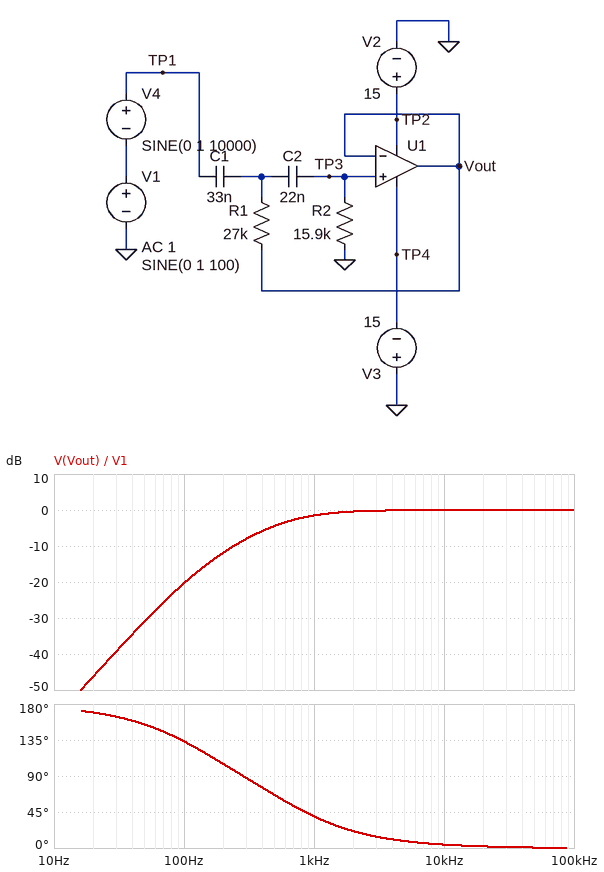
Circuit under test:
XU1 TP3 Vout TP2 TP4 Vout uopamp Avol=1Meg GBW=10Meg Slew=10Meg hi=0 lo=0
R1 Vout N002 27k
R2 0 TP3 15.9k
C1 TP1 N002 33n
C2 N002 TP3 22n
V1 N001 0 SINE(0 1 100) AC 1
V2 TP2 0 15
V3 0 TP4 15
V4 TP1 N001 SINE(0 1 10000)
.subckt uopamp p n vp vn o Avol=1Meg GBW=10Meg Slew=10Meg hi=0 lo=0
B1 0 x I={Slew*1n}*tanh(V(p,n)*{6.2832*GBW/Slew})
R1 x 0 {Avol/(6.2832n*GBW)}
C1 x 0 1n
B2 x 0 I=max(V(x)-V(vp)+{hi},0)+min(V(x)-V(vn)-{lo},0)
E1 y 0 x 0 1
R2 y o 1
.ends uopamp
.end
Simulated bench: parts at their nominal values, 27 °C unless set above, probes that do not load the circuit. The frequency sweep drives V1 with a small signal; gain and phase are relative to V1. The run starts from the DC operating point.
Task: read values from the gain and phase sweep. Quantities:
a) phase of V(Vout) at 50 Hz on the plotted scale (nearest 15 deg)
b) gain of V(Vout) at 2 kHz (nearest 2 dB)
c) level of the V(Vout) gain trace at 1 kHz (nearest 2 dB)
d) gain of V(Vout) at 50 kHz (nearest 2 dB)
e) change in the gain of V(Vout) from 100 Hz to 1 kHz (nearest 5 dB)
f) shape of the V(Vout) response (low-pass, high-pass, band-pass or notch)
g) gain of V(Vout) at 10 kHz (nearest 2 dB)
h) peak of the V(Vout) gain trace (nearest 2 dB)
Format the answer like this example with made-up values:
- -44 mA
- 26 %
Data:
- 150 deg
- 0 dB
- -2 dB
- 0 dB
- 20 dB
- high-pass
- 0 dB
- 0 dB
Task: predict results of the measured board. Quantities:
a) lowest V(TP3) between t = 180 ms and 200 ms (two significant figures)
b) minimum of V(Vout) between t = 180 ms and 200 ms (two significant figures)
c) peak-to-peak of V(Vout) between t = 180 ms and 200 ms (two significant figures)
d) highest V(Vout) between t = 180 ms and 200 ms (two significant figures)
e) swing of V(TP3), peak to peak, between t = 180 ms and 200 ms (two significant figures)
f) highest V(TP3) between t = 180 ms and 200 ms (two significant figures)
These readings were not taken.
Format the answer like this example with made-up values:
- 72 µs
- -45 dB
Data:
- -1.1 V
- -1.1 V
- 2.2 V
- 1.1 V
- 2.2 V
- 1.1 V
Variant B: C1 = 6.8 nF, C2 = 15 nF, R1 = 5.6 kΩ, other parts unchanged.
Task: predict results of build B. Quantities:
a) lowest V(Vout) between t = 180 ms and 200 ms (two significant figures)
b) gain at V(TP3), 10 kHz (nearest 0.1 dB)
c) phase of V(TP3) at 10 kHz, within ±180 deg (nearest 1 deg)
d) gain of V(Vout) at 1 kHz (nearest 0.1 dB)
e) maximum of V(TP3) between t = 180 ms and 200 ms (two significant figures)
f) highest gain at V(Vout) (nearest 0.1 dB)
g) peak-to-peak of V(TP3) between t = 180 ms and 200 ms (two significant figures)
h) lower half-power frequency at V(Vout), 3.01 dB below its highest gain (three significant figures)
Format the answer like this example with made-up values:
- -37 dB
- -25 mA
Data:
- -1.0 V
- 0 dB
- 12 deg
- -8.9 dB
- 1.0 V
- 0.1 dB
- 2.0 V
- 1.55 kHz
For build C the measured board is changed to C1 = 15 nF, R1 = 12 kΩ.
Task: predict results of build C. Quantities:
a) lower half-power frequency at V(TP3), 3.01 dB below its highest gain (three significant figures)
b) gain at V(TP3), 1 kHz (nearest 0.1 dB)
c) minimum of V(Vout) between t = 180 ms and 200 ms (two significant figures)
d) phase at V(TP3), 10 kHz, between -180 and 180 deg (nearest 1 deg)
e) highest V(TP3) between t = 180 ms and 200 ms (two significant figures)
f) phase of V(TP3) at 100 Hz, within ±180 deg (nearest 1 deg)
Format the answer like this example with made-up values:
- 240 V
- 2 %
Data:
- 830 Hz
- -2.1 dB
- -1.0 V
- 6 deg
- 1.0 V
- 164 deg
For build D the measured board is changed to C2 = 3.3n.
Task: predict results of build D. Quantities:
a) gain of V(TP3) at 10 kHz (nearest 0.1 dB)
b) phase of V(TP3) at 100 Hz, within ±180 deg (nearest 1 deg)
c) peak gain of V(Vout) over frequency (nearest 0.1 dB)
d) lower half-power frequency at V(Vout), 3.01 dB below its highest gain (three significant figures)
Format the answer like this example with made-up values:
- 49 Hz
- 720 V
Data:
- -0.4 dB
- 148 deg
- 0 dB
- 3.17 kHz
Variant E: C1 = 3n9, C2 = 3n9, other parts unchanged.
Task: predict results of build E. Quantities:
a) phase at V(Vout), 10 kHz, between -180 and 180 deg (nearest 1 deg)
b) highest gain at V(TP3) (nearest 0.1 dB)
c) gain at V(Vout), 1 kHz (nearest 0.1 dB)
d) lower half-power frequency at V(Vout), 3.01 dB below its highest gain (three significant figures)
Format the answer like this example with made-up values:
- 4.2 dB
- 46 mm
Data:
- 28 deg
- 0 dB
- -15.4 dB
- 4.40 kHz
